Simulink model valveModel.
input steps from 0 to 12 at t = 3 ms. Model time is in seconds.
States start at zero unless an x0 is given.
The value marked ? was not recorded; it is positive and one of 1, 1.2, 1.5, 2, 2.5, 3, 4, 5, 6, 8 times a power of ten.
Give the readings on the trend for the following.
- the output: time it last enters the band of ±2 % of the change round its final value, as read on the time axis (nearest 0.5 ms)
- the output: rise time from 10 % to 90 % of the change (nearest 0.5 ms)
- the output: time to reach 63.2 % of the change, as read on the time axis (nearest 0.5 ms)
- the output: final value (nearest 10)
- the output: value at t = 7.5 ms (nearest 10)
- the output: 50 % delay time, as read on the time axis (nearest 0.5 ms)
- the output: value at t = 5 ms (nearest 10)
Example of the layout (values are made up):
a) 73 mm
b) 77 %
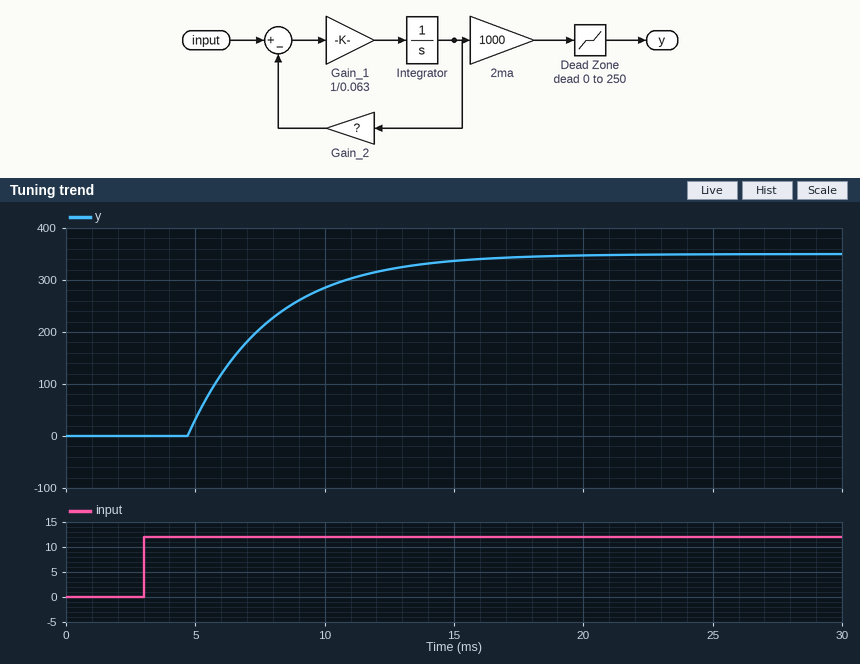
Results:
a) 17.0 ms
b) 7.0 ms
c) 8.0 ms
d) 350
e) 210
f) 7.0 ms
g) 30
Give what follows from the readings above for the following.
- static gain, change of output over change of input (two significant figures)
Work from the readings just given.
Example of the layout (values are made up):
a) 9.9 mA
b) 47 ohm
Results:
a) 29
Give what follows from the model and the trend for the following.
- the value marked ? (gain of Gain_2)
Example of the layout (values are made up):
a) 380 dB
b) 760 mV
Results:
a) 20
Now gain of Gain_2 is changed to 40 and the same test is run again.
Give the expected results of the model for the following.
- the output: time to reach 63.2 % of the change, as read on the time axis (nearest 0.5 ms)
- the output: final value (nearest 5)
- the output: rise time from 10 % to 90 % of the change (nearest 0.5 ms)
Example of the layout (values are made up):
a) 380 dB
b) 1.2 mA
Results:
a) 7.5 ms
b) 50
c) 3.5 ms
